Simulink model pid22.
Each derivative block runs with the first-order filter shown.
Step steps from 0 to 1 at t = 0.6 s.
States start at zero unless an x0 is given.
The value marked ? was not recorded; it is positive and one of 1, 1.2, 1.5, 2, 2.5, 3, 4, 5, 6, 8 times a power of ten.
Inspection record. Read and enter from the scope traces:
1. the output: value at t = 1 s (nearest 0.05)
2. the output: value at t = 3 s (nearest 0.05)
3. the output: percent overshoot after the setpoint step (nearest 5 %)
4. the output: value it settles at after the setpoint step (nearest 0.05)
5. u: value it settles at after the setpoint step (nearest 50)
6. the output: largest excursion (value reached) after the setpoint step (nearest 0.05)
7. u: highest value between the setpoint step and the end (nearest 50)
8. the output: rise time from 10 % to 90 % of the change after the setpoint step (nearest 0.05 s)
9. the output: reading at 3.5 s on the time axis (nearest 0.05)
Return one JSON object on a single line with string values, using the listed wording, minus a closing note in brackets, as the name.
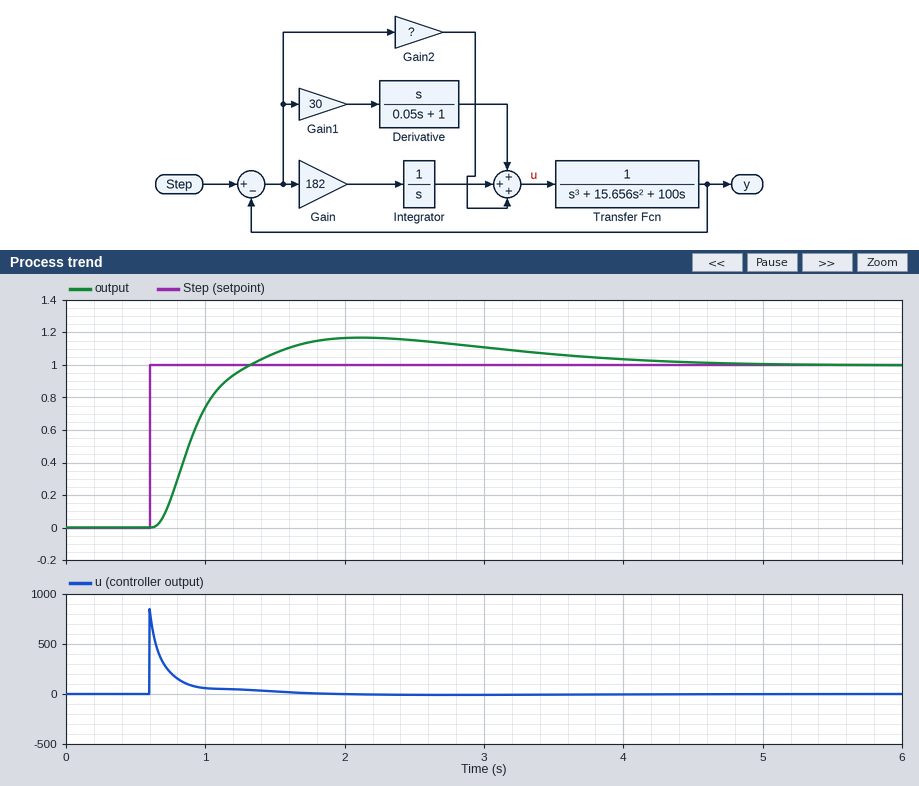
{"the output: value at t = 1 s": "0.75", "the output: value at t = 3 s": "1.10", "the output: percent overshoot after the setpoint step": "15 %", "the output: value it settles at after the setpoint step": "1.00", "u: value it settles at after the setpoint step": "0", "the output: largest excursion (value reached) after the setpoint step": "1.15", "u: highest value between the setpoint step and the end": "850", "the output: rise time from 10 % to 90 % of the change after the setpoint step": "0.45 s", "the output: reading at 3.5 s on the time axis": "1.05"}
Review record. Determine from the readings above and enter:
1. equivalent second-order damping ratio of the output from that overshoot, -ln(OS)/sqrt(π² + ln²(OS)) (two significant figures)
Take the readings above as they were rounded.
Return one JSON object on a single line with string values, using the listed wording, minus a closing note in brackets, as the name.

{"equivalent second-order damping ratio of the output from that overshoot, -ln(OS)/sqrt(π² + ln²(OS))": "0.52"}
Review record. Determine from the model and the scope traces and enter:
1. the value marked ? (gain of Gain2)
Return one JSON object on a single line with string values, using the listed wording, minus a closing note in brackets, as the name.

{"the value marked ?": "250"}
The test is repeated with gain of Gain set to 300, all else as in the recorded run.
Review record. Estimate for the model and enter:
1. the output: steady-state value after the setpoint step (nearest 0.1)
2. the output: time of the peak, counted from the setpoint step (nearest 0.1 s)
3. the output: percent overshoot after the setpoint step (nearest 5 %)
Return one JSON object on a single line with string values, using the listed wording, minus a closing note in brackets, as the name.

{"the output: steady-state value after the setpoint step": "1.0", "the output: time of the peak, counted from the setpoint step": "1.3 s", "the output: percent overshoot after the setpoint step": "25 %"}
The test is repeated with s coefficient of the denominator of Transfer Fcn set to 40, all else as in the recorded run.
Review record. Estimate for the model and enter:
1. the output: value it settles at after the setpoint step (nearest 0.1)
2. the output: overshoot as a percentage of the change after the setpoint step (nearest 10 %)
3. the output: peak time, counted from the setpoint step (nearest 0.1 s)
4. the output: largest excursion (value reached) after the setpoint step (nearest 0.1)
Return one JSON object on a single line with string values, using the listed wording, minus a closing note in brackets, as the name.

{"the output: value it settles at after the setpoint step": "1.0", "the output: overshoot as a percentage of the change after the setpoint step": "40 %", "the output: peak time, counted from the setpoint step": "0.7 s", "the output: largest excursion (value reached) after the setpoint step": "1.4"}
